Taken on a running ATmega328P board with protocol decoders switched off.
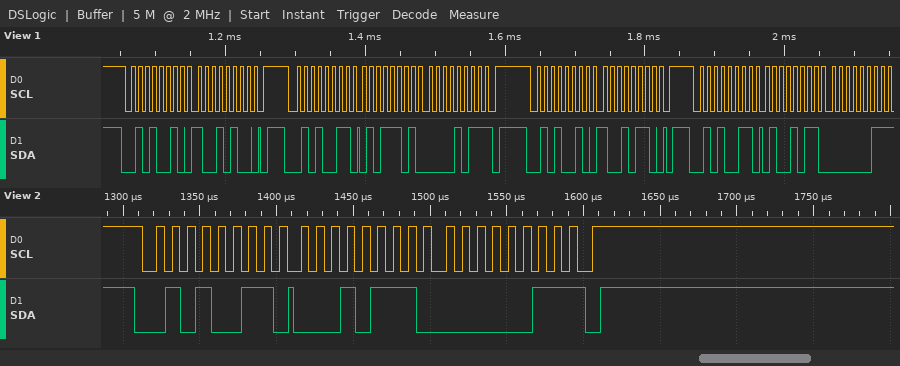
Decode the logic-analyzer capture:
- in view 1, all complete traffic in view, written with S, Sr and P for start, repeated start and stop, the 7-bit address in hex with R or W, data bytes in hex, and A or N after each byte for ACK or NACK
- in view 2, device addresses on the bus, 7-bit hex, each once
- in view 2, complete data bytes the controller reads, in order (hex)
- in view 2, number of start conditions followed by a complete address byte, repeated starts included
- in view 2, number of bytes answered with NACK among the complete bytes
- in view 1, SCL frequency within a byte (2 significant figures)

S 29W A 94 A P S 29R A 5D A 0B N P S 29W A 96 A P S 29R A 4B A 03 N
0x29
17 03
1
1
100 kHz
